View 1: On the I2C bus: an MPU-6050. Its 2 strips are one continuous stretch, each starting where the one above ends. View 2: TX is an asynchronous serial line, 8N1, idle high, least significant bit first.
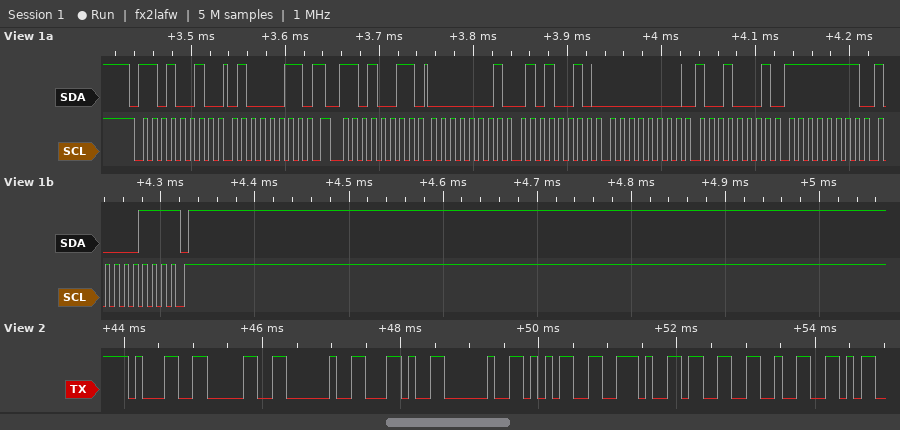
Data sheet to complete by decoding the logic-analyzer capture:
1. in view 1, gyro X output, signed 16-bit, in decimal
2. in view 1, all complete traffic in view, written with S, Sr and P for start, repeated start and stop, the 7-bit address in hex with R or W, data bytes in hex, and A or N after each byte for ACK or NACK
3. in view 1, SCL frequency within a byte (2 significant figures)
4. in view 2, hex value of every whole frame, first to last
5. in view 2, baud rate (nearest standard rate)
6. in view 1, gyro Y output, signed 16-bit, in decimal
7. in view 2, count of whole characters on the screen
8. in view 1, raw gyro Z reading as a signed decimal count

338
S 69W A 43 A Sr 69R A 01 A 52 A 00 A 91 A FF A 87 N P
100 kHz
31 30 20 2C 20 35 2E 33 32
9600 baud
145
9
-121
